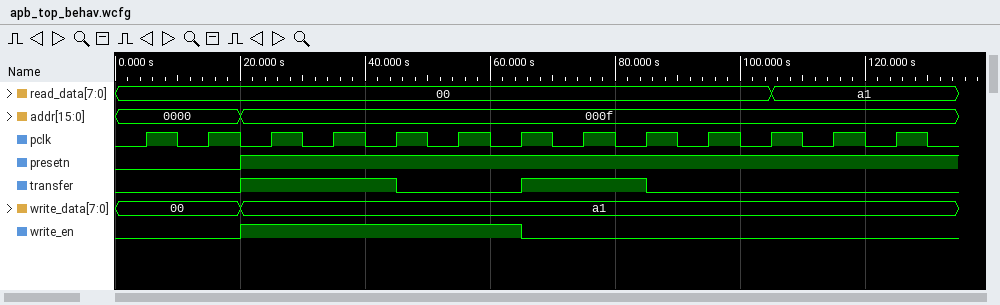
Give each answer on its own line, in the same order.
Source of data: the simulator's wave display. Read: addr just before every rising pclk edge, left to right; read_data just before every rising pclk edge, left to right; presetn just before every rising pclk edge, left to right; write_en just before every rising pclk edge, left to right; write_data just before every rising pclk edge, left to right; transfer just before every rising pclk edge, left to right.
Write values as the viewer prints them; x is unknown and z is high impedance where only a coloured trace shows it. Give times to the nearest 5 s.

0000, 0000, 000f, 000f, 000f, 000f, 000f, 000f, 000f, 000f, 000f, 000f, 000f
00, 00, 00, 00, 00, 00, 00, 00, 00, 00, 00, a1, a1
0 0 1 1 1 1 1 1 1 1 1 1 1
0 0 1 1 1 1 1 0 0 0 0 0 0
00, 00, a1, a1, a1, a1, a1, a1, a1, a1, a1, a1, a1
0 0 1 1 1 0 0 1 1 0 0 0 0
